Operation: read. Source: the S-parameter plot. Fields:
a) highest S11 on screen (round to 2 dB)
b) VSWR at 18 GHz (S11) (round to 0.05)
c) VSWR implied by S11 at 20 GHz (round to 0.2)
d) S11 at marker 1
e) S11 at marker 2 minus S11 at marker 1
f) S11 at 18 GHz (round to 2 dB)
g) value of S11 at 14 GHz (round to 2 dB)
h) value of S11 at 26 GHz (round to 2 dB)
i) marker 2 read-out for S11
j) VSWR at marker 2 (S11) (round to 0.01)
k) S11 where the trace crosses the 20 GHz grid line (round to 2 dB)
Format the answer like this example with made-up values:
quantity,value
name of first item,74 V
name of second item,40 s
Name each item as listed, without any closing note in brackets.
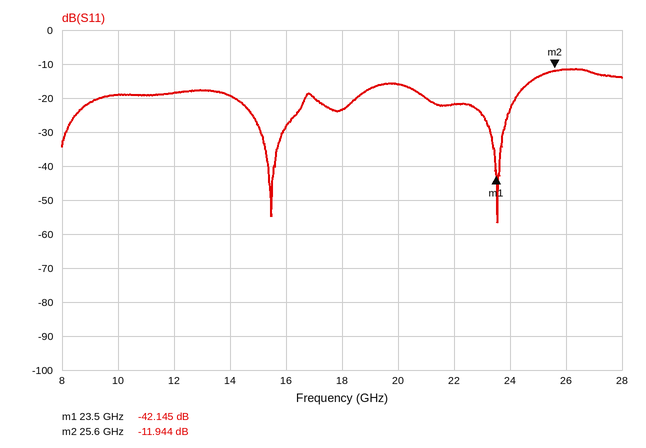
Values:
quantity,value
highest S11 on screen,-12 dB
VSWR at 18 GHz (S11),1.15
VSWR implied by S11 at 20 GHz,1.4
S11 at marker 1,-42.145 dB
S11 at marker 2 minus S11 at marker 1,30.201 dB
S11 at 18 GHz,-24 dB
value of S11 at 14 GHz,-20 dB
value of S11 at 26 GHz,-12 dB
marker 2 read-out for S11,-11.944 dB
VSWR at marker 2 (S11),1.68
S11 where the trace crosses the 20 GHz grid line,-16 dB
